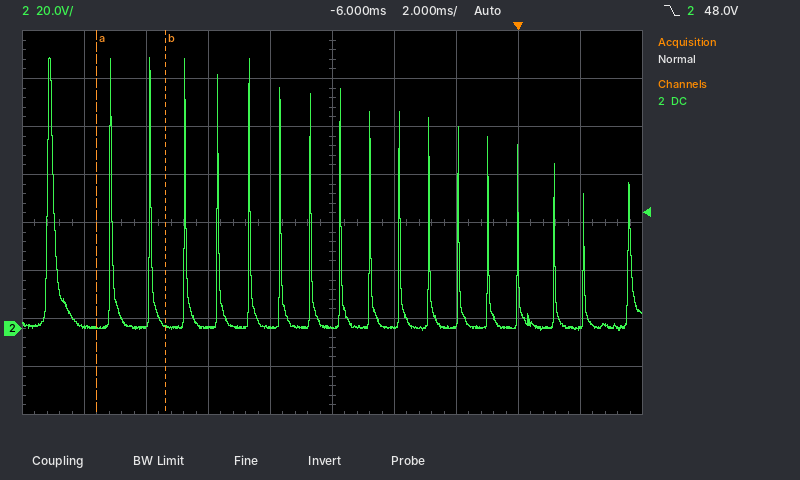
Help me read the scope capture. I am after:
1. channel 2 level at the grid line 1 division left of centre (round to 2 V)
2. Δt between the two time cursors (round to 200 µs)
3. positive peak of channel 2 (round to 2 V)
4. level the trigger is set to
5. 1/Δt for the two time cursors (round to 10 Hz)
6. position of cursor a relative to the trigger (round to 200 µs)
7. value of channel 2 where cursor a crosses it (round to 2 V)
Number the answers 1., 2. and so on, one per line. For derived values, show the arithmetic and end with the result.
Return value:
1. 0 V
2. 2.2 ms
3. 112 V
4. 48.0 V
5. 1 / 2.2 ms ≈ 450 Hz
6. -13.6 ms
7. 0 V
